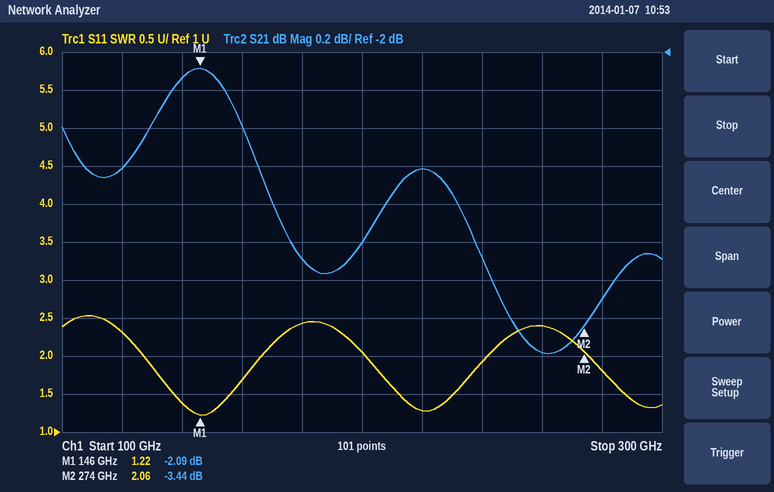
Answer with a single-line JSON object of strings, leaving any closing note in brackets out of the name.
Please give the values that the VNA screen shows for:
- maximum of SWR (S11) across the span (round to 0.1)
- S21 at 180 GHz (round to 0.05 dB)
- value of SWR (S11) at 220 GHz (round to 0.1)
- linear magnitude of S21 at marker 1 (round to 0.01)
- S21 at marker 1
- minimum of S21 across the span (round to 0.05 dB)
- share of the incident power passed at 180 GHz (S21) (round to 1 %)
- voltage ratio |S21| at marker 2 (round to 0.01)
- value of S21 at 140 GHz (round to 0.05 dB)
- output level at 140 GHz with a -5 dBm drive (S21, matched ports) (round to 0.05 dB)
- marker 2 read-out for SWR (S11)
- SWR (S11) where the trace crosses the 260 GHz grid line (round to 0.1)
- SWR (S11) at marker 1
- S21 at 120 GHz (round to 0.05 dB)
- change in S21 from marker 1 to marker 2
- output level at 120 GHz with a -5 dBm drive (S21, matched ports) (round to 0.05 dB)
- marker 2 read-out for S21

{"maximum of SWR (S11) across the span": "2.5", "S21 at 180 GHz": "-3.10 dB", "value of SWR (S11) at 220 GHz": "1.3", "linear magnitude of S21 at marker 1": "0.79", "S21 at marker 1": "-2.09 dB", "minimum of S21 across the span": "-3.60 dB", "share of the incident power passed at 180 GHz (S21)": "49 %", "voltage ratio |S21| at marker 2": "0.67", "value of S21 at 140 GHz": "-2.15 dB", "output level at 140 GHz with a -5 dBm drive (S21, matched ports)": "-7.15 dBm", "marker 2 read-out for SWR": "2.06", "SWR (S11) where the trace crosses the 260 GHz grid line": "2.4", "SWR (S11) at marker 1": "1.22", "S21 at 120 GHz": "-2.60 dB", "change in S21 from marker 1 to marker 2": "-1.35 dB", "output level at 120 GHz with a -5 dBm drive (S21, matched ports)": "-7.60 dBm", "marker 2 read-out for S21": "-3.44 dB"}
